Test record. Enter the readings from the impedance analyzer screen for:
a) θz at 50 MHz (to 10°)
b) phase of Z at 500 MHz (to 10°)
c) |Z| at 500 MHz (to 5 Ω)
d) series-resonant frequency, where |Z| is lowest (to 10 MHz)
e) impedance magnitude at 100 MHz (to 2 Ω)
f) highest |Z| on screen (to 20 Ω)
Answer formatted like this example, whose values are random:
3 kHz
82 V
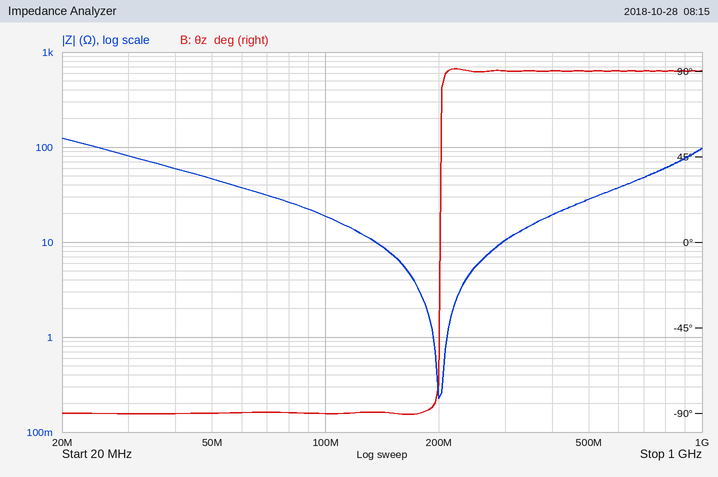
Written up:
-90°
90°
30 Ω
200 MHz
18 Ω
120 Ω
